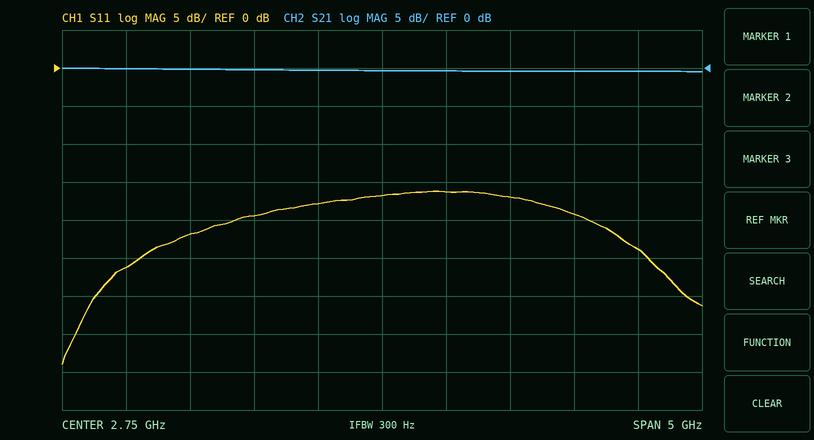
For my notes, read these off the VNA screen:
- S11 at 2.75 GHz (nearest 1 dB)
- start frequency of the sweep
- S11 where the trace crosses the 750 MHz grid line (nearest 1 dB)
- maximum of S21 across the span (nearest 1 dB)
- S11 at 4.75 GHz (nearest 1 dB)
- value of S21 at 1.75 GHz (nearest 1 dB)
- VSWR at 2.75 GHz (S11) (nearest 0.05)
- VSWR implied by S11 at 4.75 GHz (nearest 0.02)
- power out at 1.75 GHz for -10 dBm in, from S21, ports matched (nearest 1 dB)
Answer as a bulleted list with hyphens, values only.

- -17 dB
- 250 MHz
- -26 dB
- 0 dB
- -24 dB
- 0 dB
- 1.35
- 1.14
- -10 dBm
